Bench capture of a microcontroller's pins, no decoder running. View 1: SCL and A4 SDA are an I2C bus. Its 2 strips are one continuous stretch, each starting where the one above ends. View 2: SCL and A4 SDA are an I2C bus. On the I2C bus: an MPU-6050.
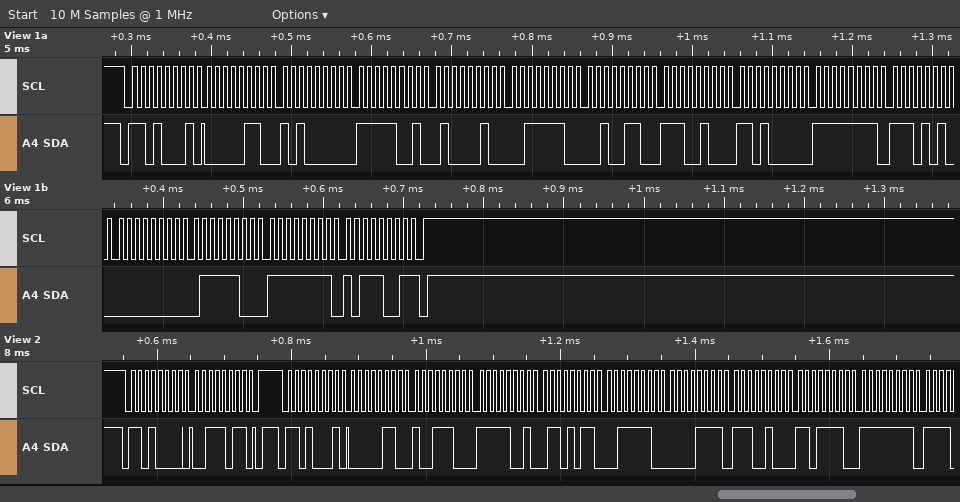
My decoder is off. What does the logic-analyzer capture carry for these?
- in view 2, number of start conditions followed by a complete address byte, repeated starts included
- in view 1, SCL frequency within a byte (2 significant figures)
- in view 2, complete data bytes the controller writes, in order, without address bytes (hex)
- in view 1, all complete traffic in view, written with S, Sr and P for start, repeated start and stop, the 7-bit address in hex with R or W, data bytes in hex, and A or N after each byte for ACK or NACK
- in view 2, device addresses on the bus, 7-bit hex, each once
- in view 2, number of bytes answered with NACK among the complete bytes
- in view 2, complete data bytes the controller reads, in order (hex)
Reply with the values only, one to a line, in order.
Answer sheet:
2
100 kHz
3B
S 68R A 06 A A0 A F9 A 42 A 3E A 26 A E4 A D0 A FF A EA A 00 A 7C A FF A B9 N P
0x68
0
06 9C F9 6B 3E 0F E4 DE FF
